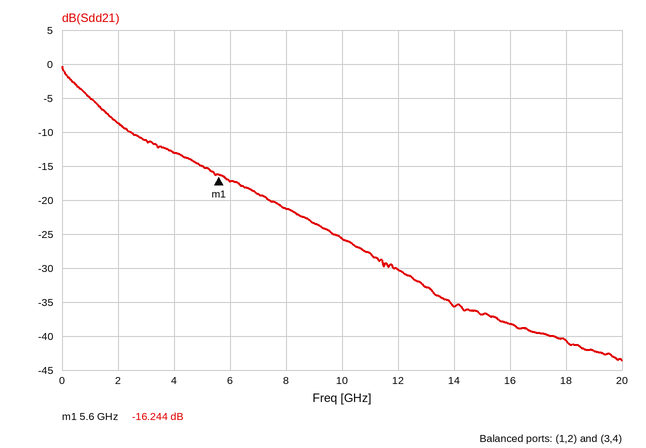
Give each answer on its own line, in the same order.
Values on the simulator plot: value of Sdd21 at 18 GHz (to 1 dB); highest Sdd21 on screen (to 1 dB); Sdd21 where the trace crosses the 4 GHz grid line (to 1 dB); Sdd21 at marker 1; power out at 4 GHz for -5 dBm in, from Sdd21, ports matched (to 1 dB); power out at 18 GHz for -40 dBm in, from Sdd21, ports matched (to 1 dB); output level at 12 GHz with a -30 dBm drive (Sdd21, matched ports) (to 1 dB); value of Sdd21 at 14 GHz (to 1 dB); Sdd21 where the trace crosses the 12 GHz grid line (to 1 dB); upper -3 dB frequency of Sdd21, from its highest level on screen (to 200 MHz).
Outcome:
-41 dB
0 dB
-13 dB
-16.244 dB
-18 dBm
-81 dBm
-60 dBm
-36 dB
-30 dB
600 MHz
